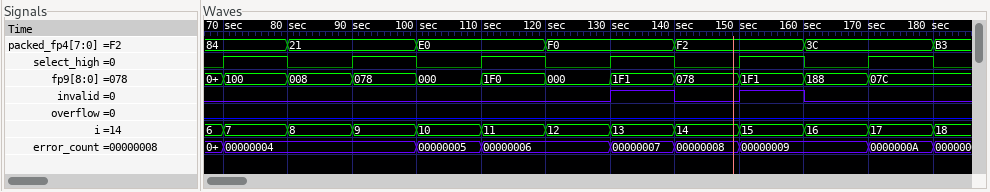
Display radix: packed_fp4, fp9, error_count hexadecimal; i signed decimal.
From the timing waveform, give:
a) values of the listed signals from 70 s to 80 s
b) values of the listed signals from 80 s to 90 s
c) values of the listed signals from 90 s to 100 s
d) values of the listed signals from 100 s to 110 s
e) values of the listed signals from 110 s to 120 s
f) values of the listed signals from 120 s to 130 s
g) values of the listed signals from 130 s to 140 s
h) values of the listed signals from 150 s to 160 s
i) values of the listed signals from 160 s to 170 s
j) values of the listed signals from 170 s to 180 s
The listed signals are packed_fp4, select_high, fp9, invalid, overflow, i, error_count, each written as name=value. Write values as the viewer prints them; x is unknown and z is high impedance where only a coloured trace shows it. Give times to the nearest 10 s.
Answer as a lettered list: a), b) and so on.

a) packed_fp4=84, select_high=1, fp9=100, invalid=0, overflow=0, i=7, error_count=00000004
b) packed_fp4=21, select_high=0, fp9=008, invalid=0, overflow=0, i=8, error_count=00000004
c) packed_fp4=21, select_high=1, fp9=078, invalid=0, overflow=0, i=9, error_count=00000004
d) packed_fp4=E0, select_high=0, fp9=000, invalid=0, overflow=0, i=10, error_count=00000005
e) packed_fp4=E0, select_high=1, fp9=1F0, invalid=0, overflow=0, i=11, error_count=00000006
f) packed_fp4=F0, select_high=0, fp9=000, invalid=0, overflow=0, i=12, error_count=00000006
g) packed_fp4=F0, select_high=1, fp9=1F1, invalid=1, overflow=0, i=13, error_count=00000007
h) packed_fp4=F2, select_high=1, fp9=1F1, invalid=1, overflow=0, i=15, error_count=00000009
i) packed_fp4=3C, select_high=0, fp9=188, invalid=0, overflow=0, i=16, error_count=00000009
j) packed_fp4=3C, select_high=1, fp9=07C, invalid=0, overflow=0, i=17, error_count=0000000A
